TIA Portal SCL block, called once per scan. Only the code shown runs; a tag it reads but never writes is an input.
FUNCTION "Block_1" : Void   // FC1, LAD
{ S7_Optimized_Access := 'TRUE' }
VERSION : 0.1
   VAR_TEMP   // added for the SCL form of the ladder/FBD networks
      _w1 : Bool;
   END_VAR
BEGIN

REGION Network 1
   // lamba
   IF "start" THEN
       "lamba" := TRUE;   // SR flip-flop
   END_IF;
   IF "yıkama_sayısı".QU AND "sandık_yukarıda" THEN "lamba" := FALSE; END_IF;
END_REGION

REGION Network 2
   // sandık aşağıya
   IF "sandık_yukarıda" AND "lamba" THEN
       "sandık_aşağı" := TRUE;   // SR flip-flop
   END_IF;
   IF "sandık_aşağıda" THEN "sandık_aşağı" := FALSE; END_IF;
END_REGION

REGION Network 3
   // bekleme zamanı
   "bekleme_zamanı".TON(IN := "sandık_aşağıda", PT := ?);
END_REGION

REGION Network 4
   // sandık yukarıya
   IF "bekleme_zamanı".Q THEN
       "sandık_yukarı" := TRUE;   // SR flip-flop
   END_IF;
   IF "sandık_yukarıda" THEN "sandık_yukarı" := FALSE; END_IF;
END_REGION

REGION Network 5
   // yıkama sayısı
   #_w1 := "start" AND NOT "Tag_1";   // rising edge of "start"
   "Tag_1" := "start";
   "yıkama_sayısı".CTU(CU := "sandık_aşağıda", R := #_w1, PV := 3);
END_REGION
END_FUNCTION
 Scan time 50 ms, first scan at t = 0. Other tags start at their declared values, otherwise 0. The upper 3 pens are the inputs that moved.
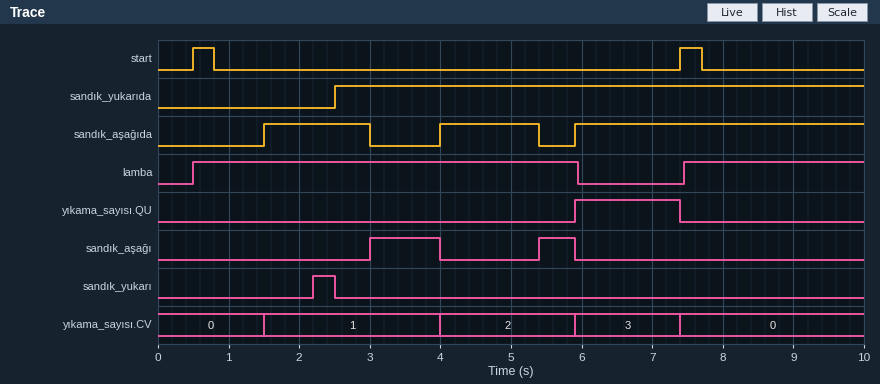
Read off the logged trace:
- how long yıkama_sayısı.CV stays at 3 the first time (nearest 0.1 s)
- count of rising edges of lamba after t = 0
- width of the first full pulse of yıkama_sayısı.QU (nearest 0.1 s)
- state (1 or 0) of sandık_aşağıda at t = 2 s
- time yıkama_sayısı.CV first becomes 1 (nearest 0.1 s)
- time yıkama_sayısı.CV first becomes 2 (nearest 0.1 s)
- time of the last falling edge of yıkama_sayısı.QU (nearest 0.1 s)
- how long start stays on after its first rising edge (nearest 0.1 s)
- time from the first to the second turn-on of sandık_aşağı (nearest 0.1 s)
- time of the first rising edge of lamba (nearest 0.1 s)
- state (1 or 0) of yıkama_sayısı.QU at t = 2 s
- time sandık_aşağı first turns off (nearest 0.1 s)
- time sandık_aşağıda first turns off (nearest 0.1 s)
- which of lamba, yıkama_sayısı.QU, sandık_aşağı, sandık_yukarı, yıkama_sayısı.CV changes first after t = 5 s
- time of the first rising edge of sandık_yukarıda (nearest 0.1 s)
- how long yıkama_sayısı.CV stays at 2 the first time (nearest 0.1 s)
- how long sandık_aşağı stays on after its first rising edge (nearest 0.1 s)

1.5 s
2
1.5 s
1
1.5 s
4.0 s
7.4 s
0.3 s
2.4 s
0.5 s
0
4.0 s
3.0 s
sandık_aşağı
2.5 s
1.9 s
1.0 s
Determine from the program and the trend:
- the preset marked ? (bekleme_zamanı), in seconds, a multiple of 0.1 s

0.7 s
